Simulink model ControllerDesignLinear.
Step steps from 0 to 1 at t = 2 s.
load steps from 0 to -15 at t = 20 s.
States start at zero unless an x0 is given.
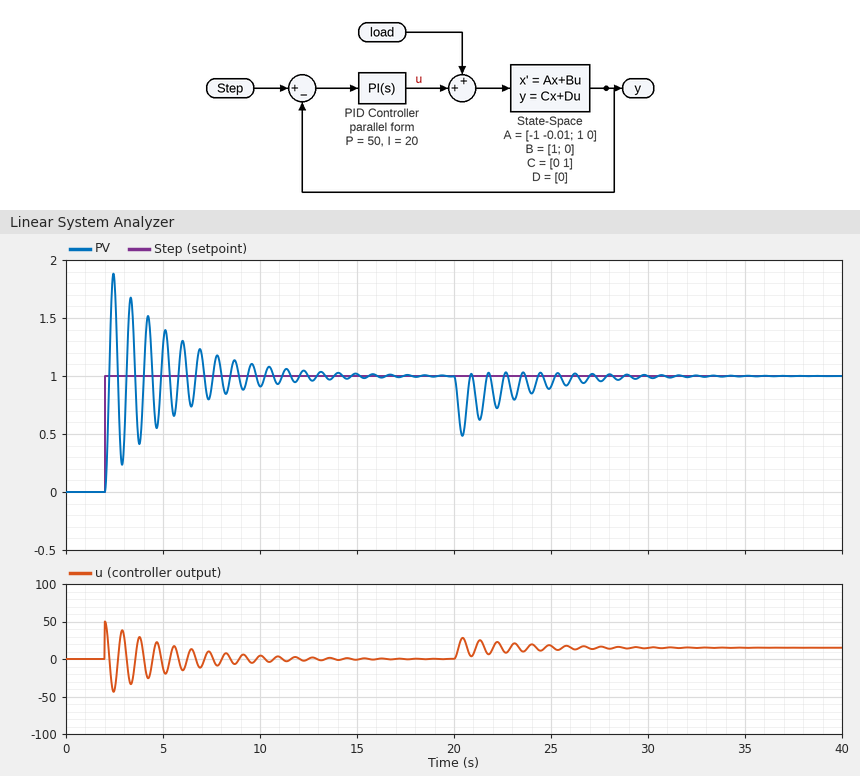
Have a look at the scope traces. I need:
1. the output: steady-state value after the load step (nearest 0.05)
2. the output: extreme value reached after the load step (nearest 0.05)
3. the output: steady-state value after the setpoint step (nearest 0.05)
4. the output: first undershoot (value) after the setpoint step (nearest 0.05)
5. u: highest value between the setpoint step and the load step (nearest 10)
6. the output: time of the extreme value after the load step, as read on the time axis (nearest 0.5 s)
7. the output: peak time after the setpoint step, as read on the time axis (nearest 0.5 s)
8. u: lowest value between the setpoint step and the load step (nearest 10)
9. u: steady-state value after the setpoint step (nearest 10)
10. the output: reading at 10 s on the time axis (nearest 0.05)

1.00
0.50
1.00
0.25
50
20.5 s
2.5 s
-40
0
0.90
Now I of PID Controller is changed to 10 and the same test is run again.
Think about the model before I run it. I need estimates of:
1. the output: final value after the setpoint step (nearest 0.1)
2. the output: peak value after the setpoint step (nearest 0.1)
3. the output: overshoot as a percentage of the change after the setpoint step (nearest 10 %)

1.0
1.8
80 %
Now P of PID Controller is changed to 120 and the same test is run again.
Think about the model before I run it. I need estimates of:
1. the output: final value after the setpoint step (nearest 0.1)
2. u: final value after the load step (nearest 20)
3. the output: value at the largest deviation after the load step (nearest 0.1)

1.0
20
0.8
